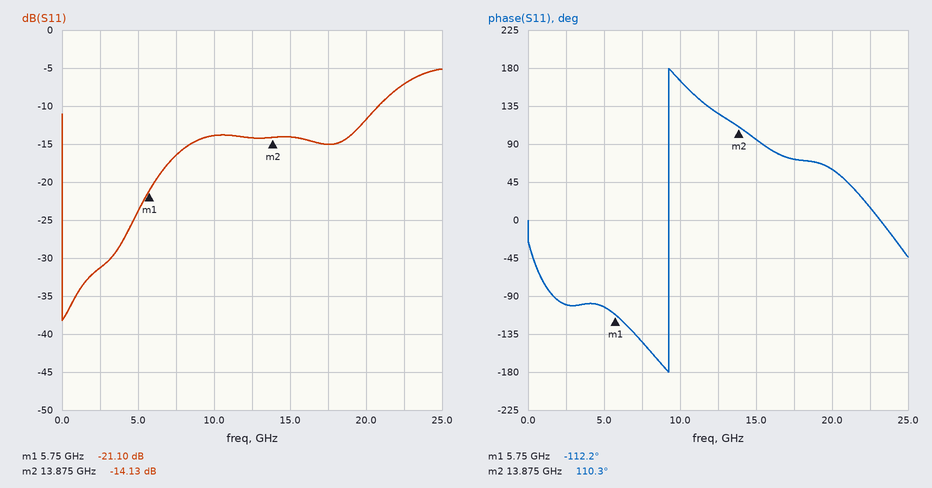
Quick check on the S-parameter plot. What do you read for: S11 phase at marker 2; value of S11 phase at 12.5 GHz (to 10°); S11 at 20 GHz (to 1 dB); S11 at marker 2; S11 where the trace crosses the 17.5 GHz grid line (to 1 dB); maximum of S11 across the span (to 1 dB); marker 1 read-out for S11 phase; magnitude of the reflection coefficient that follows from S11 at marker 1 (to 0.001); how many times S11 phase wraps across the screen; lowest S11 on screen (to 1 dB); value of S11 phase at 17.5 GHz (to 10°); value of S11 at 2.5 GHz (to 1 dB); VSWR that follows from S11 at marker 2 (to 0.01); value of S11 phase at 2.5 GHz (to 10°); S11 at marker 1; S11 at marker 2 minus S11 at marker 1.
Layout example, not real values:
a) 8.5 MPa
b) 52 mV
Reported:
a) 110.3°
b) 130°
c) -12 dB
d) -14.13 dB
e) -15 dB
f) -5 dB
g) -112.2°
h) 0.088
i) 1
j) -38 dB
k) 70°
l) -31 dB
m) 1.49
n) -100°
o) -21.10 dB
p) 6.97 dB
